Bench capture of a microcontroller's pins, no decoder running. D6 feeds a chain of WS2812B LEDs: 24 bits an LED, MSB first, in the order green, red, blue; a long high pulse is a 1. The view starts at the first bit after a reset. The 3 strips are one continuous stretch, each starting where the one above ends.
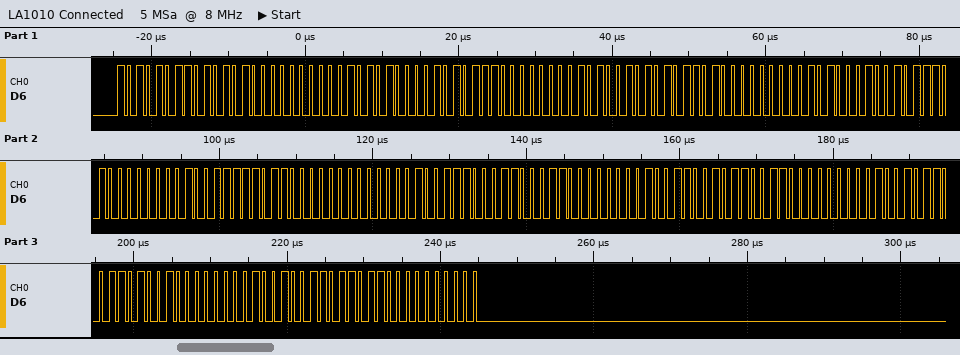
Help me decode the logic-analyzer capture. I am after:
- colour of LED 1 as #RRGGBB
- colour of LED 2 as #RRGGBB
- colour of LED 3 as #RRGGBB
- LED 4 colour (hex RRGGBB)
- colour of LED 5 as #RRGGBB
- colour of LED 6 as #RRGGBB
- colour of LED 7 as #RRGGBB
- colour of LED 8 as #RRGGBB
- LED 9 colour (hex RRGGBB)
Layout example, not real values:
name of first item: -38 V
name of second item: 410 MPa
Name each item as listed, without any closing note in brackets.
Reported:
colour of LED 1 as #RRGGBB: #54AB00
colour of LED 2 as #RRGGBB: #57A800
colour of LED 3 as #RRGGBB: #5AA500
LED 4 colour: #5DA200
colour of LED 5 as #RRGGBB: #609F00
colour of LED 6 as #RRGGBB: #639C00
colour of LED 7 as #RRGGBB: #669900
colour of LED 8 as #RRGGBB: #699600
LED 9 colour: #6C9300
